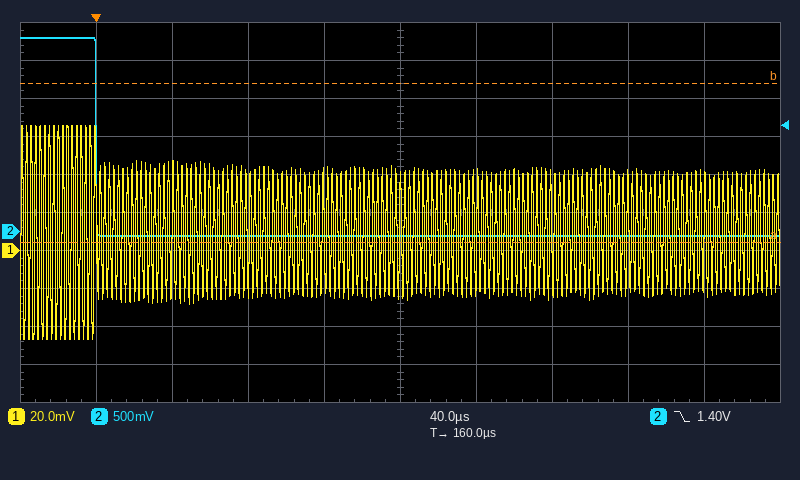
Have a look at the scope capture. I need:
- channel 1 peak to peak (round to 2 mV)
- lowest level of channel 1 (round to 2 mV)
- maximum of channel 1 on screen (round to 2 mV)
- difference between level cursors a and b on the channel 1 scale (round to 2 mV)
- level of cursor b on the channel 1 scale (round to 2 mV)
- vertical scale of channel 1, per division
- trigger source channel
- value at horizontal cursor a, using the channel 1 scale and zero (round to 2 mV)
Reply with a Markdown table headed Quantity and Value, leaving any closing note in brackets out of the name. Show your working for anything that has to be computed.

| Quantity | Value |
|---|---|
| channel 1 peak to peak | 66 mV − (-46 mV) = 112 mV |
| lowest level of channel 1 | -46 mV |
| maximum of channel 1 on screen | 66 mV |
| difference between level cursors a and b on the channel 1 scale | 84 mV |
| level of cursor b on the channel 1 scale | 88 mV |
| vertical scale of channel 1, per division | 20 mV |
| trigger source channel | channel 2 |
| value at horizontal cursor a, using the channel 1 scale and zero | 4 mV |
